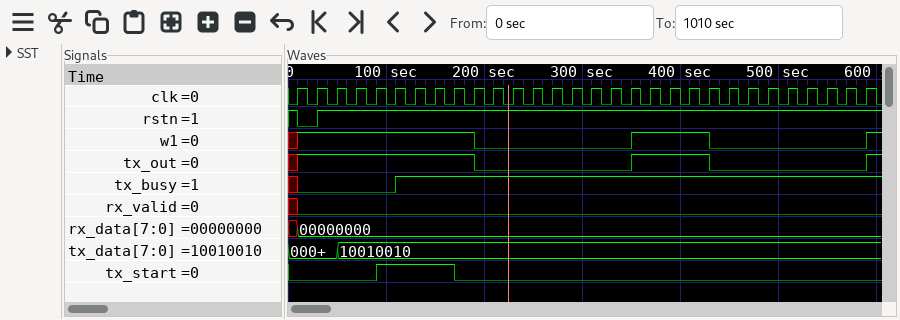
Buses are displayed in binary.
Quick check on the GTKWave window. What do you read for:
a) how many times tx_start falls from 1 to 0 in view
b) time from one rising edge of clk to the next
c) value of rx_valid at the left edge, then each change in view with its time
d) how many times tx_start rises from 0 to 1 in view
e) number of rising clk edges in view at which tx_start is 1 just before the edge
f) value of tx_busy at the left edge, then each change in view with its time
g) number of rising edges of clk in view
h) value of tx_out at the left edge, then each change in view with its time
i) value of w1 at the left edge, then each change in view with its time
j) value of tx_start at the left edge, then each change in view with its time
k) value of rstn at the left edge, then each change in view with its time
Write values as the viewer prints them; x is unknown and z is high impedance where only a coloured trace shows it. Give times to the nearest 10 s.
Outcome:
1
20 s
x, 0 at 10 s
1
4
x, 0 at 10 s, 1 at 110 s
30
x, 1 at 10 s, 0 at 190 s, 1 at 350 s, 0 at 430 s, 1 at 590 s
x, 1 at 10 s, 0 at 190 s, 1 at 350 s, 0 at 430 s, 1 at 590 s
0, 1 at 90 s, 0 at 170 s
1, 0 at 10 s, 1 at 30 s
